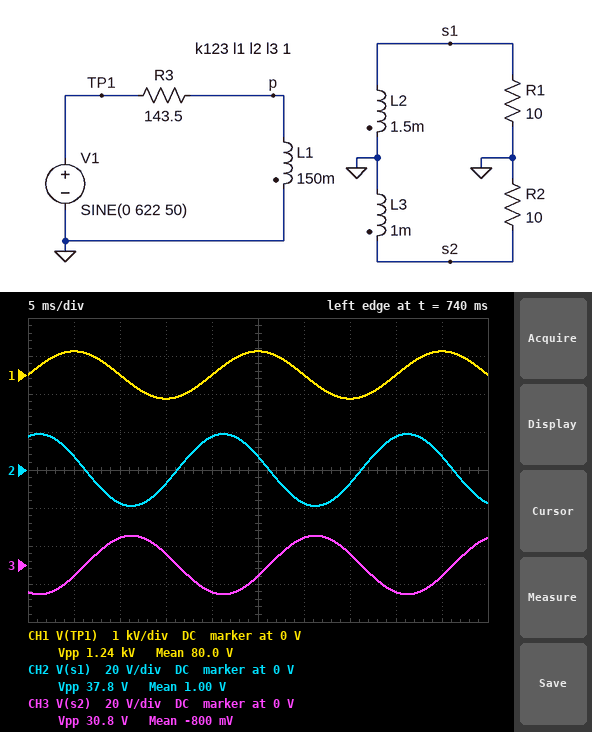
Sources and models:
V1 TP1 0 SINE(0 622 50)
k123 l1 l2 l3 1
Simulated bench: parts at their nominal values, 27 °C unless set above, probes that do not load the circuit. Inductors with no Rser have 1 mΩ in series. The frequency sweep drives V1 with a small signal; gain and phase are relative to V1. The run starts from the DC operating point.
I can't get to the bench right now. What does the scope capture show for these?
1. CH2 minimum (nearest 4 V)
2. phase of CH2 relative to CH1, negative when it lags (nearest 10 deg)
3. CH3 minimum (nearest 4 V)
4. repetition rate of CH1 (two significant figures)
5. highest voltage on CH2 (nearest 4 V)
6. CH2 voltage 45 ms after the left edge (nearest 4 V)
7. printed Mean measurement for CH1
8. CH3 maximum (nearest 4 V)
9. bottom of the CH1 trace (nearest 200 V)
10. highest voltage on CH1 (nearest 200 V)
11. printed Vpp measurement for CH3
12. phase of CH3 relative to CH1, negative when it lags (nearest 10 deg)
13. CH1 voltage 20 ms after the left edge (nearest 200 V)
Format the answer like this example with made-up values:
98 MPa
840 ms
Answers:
-20 V
70 deg
-16 V
50 Hz
20 V
8 V
80.0 V
16 V
-600 V
600 V
30.8 V
-110 deg
0 V
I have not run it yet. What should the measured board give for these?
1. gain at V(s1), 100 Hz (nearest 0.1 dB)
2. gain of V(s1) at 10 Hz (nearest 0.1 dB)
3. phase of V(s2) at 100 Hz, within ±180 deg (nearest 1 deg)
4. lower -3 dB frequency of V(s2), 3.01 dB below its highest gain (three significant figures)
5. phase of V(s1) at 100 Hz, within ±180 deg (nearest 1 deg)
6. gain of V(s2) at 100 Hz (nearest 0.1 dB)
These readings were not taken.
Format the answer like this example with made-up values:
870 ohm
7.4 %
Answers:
-25.9 dB
-43.7 dB
-129 deg
123 Hz
51 deg
-27.6 dB
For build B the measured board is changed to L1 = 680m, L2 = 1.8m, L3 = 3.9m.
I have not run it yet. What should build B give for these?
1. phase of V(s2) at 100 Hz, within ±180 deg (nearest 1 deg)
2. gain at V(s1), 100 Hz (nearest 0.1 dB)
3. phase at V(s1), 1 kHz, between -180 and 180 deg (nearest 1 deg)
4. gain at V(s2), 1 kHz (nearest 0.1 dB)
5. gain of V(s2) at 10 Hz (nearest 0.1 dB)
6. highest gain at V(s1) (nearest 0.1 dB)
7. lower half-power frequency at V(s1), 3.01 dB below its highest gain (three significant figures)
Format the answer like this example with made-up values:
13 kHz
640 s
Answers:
-163 deg
-27.1 dB
2 deg
-23.4 dB
-33.4 dB
-26.8 dB
30.0 Hz
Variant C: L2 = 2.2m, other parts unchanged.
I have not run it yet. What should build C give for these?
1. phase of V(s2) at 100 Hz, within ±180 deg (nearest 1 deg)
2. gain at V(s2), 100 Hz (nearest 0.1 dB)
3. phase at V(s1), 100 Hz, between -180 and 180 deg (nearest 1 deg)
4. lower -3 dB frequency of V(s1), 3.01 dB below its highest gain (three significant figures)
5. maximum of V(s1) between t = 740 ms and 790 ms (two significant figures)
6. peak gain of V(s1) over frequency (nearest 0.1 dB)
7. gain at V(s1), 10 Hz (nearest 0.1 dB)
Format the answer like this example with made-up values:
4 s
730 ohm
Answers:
-131 deg
-27.8 dB
49 deg
117 Hz
23 V
-20.7 dB
-42.0 dB
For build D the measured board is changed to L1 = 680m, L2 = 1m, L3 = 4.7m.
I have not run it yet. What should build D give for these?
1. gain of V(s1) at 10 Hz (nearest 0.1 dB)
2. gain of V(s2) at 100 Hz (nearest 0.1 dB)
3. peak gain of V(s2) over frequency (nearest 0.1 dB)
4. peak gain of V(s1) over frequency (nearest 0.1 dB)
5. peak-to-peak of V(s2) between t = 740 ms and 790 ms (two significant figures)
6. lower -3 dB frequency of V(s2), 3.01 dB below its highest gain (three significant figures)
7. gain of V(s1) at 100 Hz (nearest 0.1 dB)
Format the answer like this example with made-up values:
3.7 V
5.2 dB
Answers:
-39.3 dB
-23.0 dB
-22.6 dB
-29.3 dB
79 V
30.0 Hz
-29.7 dB
